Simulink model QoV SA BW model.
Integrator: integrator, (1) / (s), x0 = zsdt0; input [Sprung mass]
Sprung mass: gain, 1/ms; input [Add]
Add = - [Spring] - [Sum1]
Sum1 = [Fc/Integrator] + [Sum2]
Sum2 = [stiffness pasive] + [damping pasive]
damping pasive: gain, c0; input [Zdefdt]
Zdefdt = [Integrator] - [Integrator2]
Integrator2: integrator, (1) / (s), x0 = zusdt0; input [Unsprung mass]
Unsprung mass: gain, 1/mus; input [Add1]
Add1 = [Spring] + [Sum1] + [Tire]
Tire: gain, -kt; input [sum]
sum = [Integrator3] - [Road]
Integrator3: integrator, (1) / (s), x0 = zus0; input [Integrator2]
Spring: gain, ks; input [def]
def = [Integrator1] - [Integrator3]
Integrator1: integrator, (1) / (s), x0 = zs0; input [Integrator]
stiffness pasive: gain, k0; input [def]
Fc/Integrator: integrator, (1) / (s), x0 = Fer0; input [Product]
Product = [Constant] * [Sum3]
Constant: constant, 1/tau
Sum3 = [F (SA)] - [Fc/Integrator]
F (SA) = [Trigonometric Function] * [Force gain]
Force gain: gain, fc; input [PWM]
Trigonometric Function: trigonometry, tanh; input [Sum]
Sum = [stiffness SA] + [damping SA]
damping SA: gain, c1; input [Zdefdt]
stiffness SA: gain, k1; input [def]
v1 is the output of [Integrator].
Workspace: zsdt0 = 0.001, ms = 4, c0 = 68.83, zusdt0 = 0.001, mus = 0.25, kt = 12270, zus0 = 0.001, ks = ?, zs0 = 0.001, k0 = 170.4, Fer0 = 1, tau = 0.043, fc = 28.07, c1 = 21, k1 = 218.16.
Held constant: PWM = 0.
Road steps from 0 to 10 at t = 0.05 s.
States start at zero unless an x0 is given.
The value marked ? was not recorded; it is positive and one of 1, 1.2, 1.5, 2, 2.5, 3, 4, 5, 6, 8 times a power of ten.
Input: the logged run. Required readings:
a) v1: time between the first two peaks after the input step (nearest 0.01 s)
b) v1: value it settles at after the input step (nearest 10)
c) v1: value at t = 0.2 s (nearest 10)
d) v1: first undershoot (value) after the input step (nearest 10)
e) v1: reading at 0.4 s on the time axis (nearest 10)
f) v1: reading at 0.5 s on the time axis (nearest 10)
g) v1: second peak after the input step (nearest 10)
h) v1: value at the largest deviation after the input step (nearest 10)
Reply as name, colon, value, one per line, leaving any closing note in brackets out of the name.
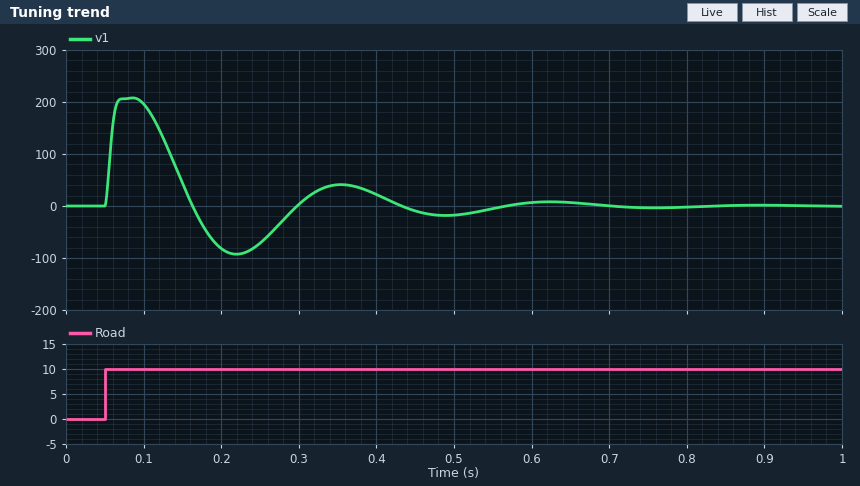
v1: time between the first two peaks after the input step: 0.27 s
v1: value it settles at after the input step: 0
v1: value at t = 0.2 s: -80
v1: first undershoot (value) after the input step: -90
v1: reading at 0.4 s on the time axis: 20
v1: reading at 0.5 s on the time axis: -20
v1: second peak after the input step: 40
v1: value at the largest deviation after the input step: 210
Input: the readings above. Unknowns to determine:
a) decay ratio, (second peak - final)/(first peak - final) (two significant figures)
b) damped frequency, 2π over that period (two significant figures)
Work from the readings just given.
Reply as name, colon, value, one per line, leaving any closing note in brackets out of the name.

decay ratio, (second peak - final)/(first peak - final): 0.19
damped frequency, 2π over that period: 23 rad/s
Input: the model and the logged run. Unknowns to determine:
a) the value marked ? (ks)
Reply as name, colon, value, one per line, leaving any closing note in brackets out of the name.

the value marked ?: 2500
